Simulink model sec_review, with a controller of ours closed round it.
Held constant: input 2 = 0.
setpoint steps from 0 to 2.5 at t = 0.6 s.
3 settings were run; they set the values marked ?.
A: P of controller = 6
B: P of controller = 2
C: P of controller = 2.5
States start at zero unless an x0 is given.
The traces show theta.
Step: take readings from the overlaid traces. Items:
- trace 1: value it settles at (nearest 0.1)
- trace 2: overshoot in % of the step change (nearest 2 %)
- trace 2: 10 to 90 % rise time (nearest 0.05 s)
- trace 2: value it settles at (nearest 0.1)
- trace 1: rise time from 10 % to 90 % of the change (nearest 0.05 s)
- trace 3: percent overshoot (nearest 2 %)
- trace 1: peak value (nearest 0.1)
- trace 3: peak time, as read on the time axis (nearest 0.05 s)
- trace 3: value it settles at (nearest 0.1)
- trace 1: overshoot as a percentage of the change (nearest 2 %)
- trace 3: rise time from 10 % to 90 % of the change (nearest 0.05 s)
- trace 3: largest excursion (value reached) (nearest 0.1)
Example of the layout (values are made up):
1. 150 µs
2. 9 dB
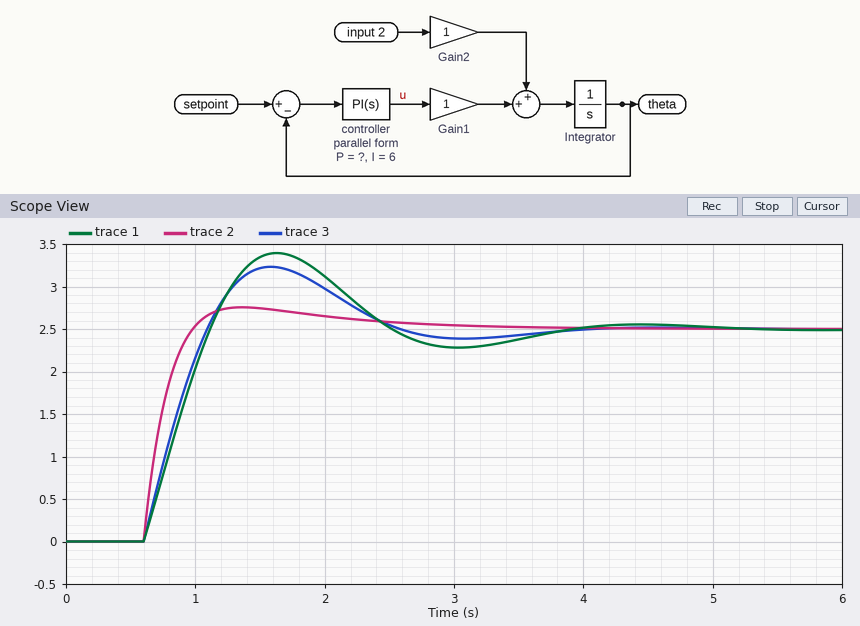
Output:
1. 2.5
2. 10 %
3. 0.25 s
4. 2.5
5. 0.40 s
6. 30 %
7. 3.4
8. 1.60 s
9. 2.5
10. 36 %
11. 0.40 s
12. 3.2
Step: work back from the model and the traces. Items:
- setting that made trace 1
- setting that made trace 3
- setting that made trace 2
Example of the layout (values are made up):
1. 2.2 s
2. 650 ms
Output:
1. B
2. C
3. A
